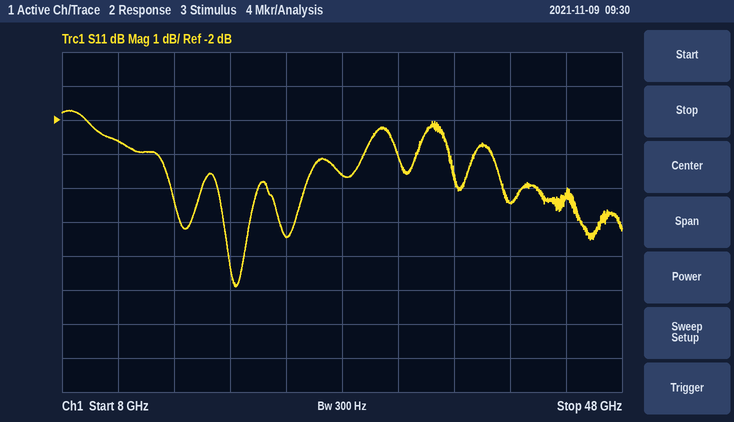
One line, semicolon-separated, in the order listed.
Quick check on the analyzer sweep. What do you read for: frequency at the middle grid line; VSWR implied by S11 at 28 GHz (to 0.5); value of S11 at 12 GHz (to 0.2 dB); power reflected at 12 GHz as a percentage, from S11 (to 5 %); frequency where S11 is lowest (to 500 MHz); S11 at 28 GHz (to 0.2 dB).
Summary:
28 GHz; 5.0; -2.6 dB; 55 %; 20.5 GHz; -3.6 dB
